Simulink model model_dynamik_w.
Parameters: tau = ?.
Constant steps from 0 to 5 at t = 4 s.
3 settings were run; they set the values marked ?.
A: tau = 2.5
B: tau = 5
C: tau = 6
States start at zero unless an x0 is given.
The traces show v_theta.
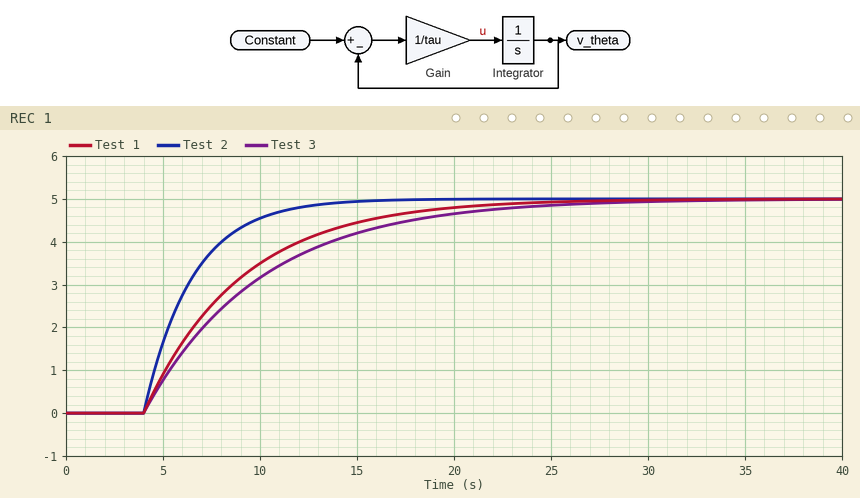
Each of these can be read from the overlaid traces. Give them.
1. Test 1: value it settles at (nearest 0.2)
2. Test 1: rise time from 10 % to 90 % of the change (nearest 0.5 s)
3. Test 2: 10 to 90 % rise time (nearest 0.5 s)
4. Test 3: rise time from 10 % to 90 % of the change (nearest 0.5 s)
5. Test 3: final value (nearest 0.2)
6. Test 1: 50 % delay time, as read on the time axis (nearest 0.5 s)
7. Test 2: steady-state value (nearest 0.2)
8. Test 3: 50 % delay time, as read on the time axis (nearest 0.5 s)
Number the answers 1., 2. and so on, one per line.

1. 5.0
2. 11.0 s
3. 5.5 s
4. 13.0 s
5. 5.0
6. 7.5 s
7. 5.0
8. 8.0 s
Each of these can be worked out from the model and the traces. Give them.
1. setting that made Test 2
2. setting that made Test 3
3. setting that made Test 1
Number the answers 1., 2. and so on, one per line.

1. A
2. C
3. B
